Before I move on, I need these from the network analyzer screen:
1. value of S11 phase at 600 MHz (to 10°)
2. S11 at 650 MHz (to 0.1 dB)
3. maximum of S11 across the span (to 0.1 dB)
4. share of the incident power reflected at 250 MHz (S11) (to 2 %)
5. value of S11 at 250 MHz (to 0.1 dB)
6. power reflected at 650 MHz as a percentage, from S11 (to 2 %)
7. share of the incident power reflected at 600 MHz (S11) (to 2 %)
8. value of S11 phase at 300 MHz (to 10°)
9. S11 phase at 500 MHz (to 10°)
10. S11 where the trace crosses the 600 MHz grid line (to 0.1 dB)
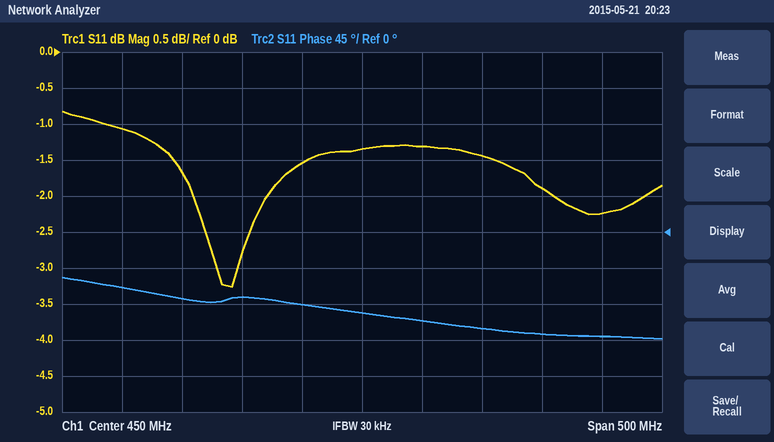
-130°
-2.2 dB
-0.8 dB
78 %
-1.1 dB
60 %
64 %
-80°
-110°
-1.9 dB
